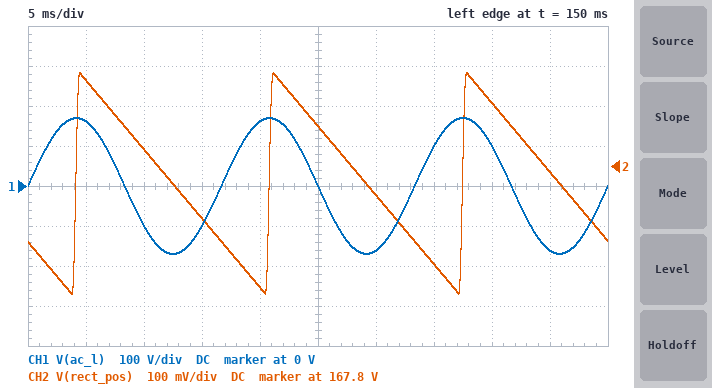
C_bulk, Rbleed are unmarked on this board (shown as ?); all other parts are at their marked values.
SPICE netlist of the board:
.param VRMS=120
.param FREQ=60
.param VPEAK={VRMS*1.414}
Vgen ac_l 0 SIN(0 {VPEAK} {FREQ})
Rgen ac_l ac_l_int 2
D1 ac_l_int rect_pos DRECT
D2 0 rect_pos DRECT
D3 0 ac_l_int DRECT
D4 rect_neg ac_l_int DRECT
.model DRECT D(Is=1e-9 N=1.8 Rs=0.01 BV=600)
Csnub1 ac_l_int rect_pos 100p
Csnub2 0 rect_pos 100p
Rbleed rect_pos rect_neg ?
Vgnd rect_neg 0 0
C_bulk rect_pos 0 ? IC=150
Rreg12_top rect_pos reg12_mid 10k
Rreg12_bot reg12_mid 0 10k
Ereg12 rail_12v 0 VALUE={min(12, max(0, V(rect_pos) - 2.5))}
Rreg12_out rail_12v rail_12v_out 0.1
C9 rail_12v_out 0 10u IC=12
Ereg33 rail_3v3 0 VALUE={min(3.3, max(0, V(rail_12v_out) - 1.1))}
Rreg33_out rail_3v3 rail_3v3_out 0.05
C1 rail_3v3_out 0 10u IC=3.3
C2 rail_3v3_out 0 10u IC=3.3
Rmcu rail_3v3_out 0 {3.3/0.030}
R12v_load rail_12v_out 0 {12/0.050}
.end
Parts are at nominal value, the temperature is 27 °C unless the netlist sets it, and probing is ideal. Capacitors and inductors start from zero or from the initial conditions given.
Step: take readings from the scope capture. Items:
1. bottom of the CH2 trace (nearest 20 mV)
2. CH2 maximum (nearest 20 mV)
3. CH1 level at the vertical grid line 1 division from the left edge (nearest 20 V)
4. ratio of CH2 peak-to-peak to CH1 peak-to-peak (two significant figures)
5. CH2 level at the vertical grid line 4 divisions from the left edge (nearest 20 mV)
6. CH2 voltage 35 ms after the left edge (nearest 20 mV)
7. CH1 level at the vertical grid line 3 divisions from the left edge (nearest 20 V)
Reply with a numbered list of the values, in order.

1. 167.48 V
2. 168.04 V
3. 160 V
4. 0.0016
5. 167.50 V
6. 167.56 V
7. -100 V
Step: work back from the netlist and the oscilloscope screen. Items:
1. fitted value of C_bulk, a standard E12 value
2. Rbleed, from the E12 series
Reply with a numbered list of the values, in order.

1. 330 µF
2. 56 kΩ
